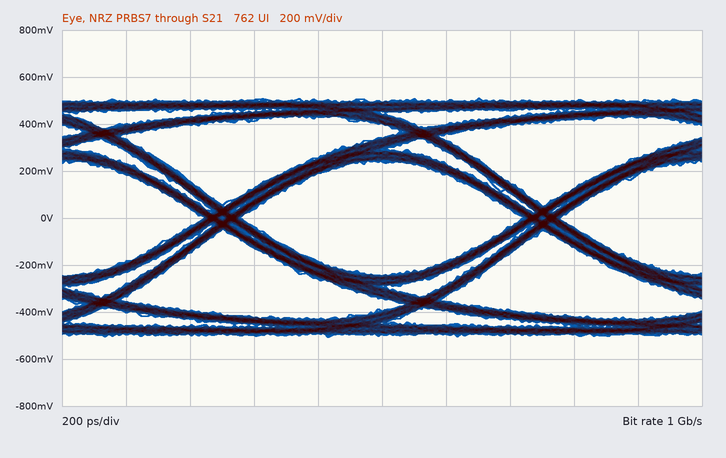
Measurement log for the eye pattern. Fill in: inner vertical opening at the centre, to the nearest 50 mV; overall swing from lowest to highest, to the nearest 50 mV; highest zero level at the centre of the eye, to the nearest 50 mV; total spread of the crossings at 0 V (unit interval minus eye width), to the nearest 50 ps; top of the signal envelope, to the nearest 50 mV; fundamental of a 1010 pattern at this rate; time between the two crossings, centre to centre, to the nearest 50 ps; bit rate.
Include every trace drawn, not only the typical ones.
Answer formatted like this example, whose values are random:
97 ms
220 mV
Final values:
500 mV
1.00 V
-250 mV
100 ps
500 mV
500 MHz
1.00 ns
1 Gb/s
